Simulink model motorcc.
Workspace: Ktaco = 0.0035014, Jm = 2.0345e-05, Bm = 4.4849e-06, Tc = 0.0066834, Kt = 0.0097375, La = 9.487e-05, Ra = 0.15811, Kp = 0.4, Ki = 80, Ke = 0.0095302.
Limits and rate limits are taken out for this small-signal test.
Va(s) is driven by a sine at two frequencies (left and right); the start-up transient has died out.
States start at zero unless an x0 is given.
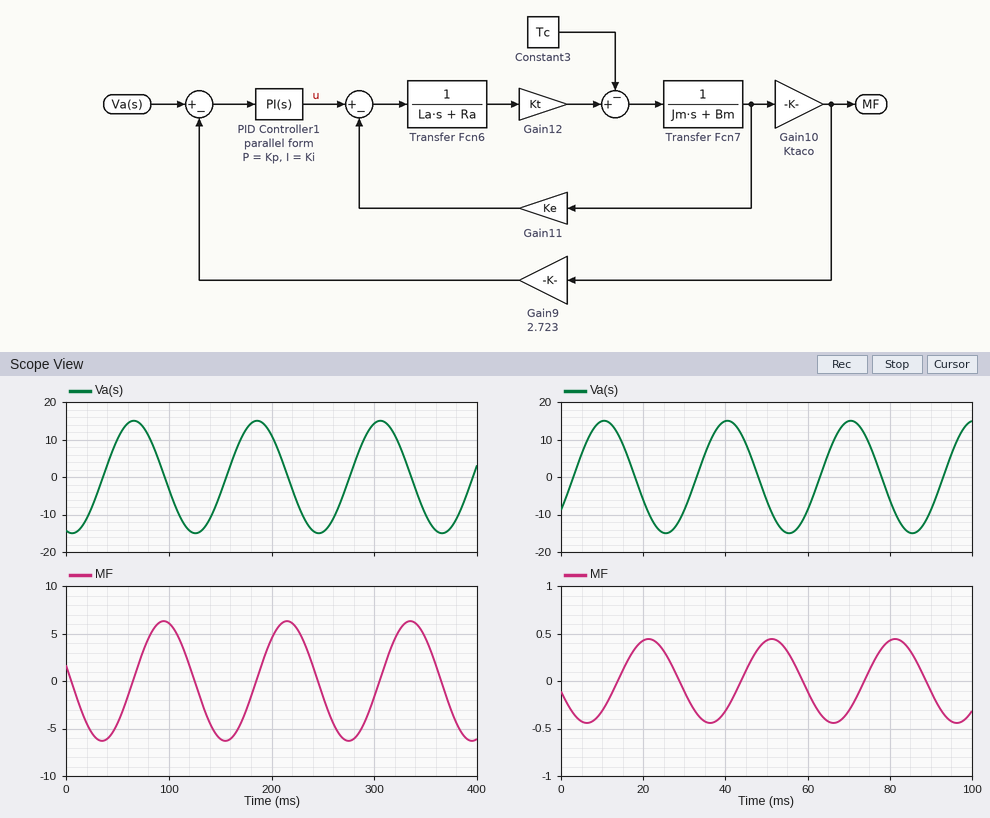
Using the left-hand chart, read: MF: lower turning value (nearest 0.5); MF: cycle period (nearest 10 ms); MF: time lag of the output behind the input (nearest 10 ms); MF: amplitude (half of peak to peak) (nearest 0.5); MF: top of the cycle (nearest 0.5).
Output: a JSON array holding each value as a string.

["-6.5", "120 ms", "30 ms", "6.5", "6.5"]
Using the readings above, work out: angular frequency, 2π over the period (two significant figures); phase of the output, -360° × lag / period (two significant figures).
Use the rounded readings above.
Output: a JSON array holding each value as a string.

["0.052 rad/ms", "-90°"]
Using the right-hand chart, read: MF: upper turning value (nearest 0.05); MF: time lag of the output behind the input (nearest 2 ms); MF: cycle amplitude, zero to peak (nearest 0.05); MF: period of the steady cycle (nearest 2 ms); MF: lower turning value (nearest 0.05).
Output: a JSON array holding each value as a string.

["0.45", "10 ms", "0.45", "30 ms", "-0.45"]
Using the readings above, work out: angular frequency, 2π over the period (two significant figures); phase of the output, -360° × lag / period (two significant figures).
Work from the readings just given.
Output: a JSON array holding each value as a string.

["0.21 rad/ms", "-120°"]
